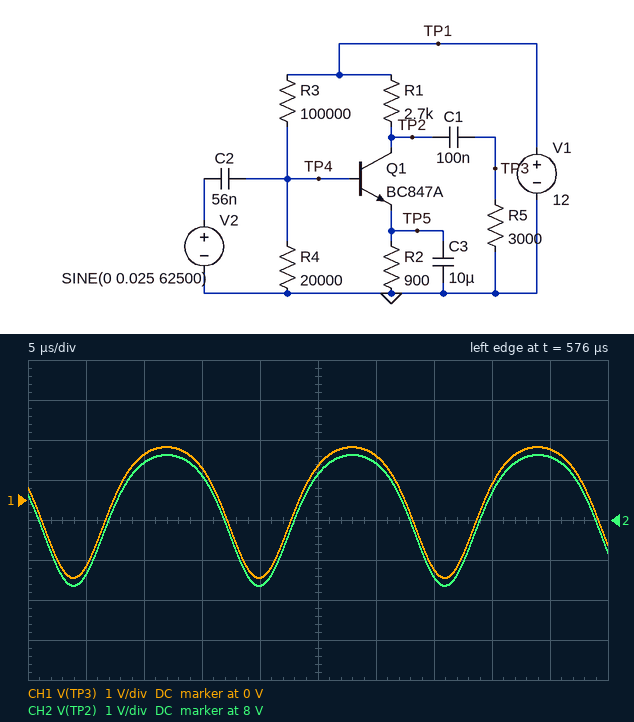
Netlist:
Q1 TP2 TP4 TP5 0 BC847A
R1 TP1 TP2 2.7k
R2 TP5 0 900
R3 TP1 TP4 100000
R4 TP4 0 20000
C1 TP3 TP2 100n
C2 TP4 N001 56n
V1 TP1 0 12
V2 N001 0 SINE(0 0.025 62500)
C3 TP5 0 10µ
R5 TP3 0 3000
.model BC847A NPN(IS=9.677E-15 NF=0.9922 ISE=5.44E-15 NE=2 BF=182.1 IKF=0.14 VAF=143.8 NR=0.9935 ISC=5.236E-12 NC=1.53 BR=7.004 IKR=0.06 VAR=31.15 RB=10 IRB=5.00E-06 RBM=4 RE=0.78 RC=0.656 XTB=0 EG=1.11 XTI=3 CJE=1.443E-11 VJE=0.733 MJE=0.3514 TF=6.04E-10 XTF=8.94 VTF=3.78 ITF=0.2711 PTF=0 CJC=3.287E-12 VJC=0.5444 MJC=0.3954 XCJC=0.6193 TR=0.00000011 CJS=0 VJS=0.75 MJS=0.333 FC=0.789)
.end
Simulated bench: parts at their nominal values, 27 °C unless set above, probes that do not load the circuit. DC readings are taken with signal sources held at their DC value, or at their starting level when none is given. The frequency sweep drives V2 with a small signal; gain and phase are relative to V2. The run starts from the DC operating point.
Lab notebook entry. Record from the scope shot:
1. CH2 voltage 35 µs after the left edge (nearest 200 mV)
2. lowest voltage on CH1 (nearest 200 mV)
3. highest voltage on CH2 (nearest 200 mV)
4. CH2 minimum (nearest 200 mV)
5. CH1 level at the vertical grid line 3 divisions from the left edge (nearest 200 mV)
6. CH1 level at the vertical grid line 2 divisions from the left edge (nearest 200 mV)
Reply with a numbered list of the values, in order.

1. 6.6 V
2. -2.0 V
3. 9.6 V
4. 6.4 V
5. 800 mV
6. 1.2 V
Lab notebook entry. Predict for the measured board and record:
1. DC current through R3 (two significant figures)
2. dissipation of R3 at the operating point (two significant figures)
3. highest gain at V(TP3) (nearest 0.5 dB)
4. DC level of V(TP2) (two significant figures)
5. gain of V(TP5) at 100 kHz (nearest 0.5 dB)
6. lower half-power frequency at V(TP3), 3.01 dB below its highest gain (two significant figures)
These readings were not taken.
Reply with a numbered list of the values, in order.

1. 100 µA
2. 1.0 mW
3. 37.0 dB
4. 8.4 V
5. -42.0 dB
6. 1.7 kHz
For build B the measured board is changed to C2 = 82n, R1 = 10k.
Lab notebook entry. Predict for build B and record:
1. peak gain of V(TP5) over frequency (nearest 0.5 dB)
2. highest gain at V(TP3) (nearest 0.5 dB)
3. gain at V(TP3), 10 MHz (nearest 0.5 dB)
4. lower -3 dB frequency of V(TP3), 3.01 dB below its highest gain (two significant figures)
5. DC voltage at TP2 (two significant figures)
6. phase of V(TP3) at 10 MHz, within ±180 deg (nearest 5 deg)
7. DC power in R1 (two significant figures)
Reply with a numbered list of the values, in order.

1. -36.5 dB
2. 24.5 dB
3. 10.0 dB
4. 15 kHz
5. 1.1 V
6. 85 deg
7. 12 mW
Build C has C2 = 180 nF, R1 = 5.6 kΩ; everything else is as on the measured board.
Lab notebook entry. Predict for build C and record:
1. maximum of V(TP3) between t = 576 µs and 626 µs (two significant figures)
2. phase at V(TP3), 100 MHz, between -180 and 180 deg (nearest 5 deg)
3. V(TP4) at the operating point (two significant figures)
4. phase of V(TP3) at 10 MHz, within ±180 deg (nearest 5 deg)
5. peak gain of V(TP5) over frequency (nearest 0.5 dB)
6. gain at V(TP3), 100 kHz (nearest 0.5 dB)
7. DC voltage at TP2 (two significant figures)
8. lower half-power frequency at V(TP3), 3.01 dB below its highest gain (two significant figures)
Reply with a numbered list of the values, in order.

1. 1.8 V
2. 100 deg
3. 1.9 V
4. 165 deg
5. -3.0 dB
6. 39.5 dB
7. 4.5 V
8. 1.1 kHz
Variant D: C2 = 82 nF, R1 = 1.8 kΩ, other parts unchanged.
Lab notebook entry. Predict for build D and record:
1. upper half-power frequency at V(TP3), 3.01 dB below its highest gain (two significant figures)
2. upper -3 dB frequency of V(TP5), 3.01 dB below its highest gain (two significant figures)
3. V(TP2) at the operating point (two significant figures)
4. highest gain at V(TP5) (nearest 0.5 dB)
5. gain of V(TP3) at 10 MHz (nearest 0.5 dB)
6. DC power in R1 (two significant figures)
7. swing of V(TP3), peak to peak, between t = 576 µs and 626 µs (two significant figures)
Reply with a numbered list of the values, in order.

1. 95 MHz
2. 1.5 kHz
3. 9.6 V
4. -5.5 dB
5. 35.0 dB
6. 3.3 mW
7. 2.6 V
